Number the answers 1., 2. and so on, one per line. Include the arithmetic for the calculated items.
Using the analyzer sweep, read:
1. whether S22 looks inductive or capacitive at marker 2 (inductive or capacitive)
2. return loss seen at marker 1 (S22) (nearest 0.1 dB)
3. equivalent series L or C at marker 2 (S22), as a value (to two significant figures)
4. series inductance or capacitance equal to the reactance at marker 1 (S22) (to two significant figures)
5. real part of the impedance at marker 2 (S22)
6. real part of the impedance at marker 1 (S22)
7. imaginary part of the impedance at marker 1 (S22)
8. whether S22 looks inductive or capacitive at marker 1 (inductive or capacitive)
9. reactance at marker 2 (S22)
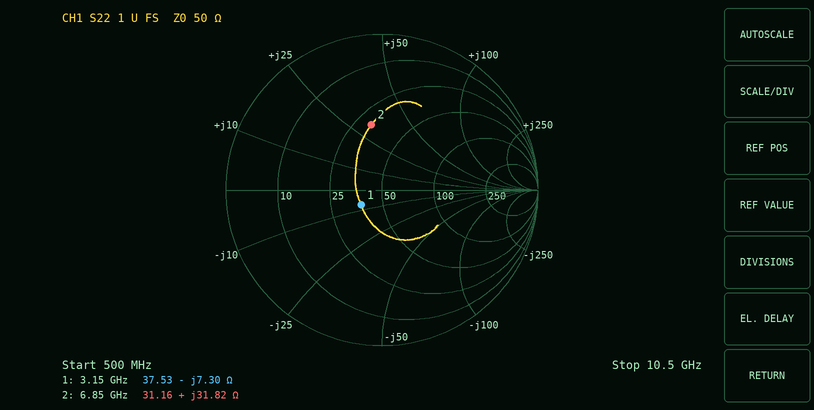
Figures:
1. inductive
2. 15.7 dB
3. L = 31.82 Ω/(2π × 6.85 GHz) ≈ 739 pH, so 740 pH to two significant figures
4. C = 1/(2π × 3.15 GHz × 7.3 Ω) ≈ 6.9 pF
5. 31.16 Ω
6. 37.53 Ω
7. -7.30 Ω
8. capacitive
9. +31.82 Ω
